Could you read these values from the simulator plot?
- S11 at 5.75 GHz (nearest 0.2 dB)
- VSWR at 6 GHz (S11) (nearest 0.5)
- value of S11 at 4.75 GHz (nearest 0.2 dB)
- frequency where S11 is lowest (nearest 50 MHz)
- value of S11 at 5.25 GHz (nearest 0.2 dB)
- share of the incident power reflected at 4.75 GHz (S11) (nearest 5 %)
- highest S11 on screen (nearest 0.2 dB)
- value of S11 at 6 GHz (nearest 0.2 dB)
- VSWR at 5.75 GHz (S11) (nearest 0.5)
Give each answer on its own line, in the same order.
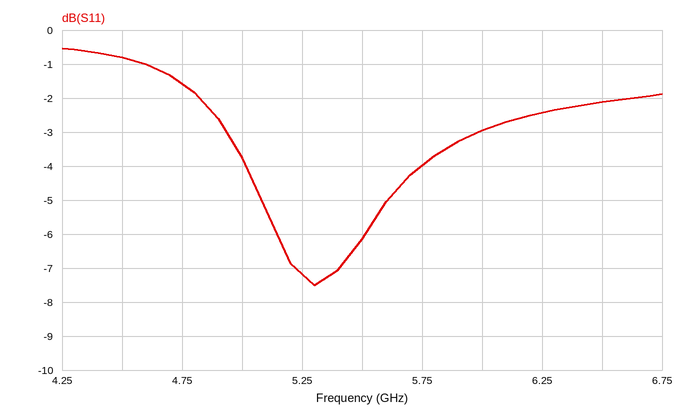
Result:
-4.0 dB
6.0
-1.6 dB
5.30 GHz
-7.2 dB
70 %
-0.6 dB
-3.0 dB
4.5
